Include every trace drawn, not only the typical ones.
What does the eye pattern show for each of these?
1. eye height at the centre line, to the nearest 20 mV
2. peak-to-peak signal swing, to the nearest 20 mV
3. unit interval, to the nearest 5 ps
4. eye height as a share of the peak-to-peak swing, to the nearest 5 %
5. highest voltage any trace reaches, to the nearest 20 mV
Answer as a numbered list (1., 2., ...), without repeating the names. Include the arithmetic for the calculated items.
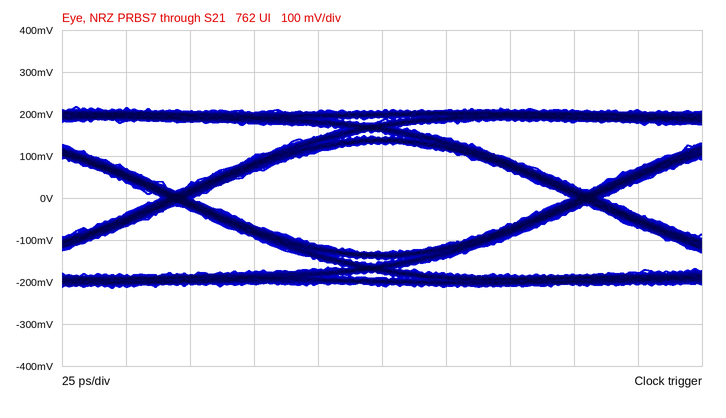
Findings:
1. 260 mV
2. 440 mV
3. 160 ps
4. 260 mV / 440 mV ≈ 59.1 %, so 60 % to the nearest 5 %
5. 220 mV
